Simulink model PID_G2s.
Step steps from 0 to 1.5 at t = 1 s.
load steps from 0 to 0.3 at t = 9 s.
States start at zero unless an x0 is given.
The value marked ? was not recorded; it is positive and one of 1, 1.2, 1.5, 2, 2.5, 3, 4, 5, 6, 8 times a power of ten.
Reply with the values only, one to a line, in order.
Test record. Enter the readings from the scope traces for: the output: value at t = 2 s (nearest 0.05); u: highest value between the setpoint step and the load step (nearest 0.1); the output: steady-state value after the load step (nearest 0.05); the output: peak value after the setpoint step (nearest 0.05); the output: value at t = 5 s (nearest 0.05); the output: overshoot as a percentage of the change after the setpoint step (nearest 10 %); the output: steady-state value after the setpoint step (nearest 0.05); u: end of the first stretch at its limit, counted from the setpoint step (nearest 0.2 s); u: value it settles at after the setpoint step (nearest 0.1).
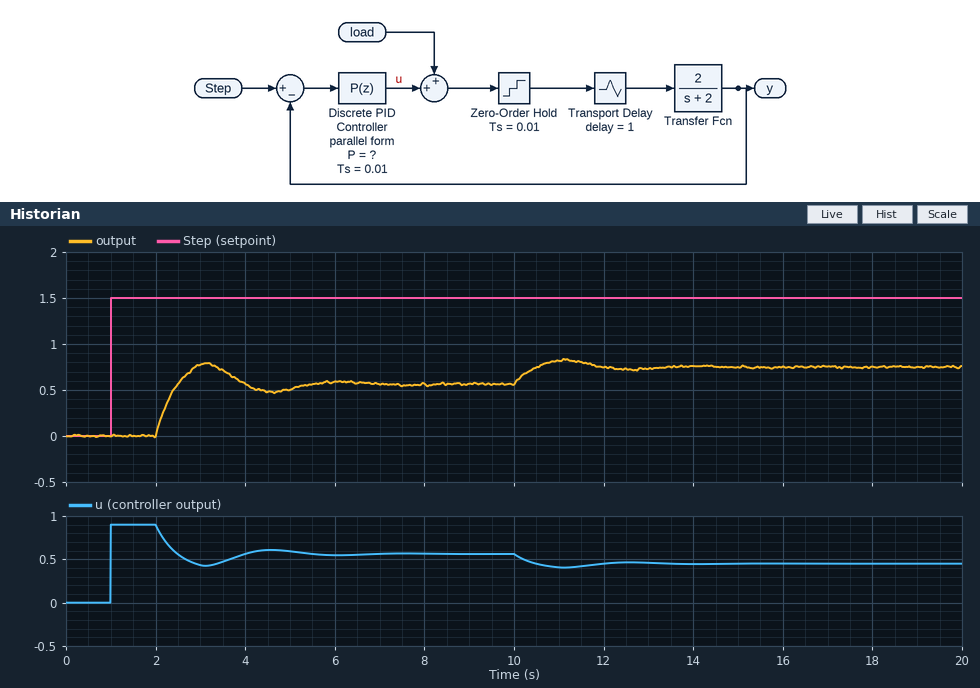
0.00
0.9
0.75
0.80
0.50
40 %
0.55
1.0 s
0.6
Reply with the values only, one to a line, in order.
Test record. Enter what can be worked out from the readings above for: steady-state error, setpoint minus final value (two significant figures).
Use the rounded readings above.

0.95
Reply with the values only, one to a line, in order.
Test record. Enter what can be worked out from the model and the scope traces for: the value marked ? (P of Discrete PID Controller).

0.6
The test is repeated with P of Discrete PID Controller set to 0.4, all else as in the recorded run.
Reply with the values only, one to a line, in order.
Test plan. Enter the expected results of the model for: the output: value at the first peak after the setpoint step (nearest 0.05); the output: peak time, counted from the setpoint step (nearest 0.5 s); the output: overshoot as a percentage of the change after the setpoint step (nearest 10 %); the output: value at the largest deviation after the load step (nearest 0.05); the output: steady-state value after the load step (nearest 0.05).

0.55
2.0 s
20 %
0.70
0.65
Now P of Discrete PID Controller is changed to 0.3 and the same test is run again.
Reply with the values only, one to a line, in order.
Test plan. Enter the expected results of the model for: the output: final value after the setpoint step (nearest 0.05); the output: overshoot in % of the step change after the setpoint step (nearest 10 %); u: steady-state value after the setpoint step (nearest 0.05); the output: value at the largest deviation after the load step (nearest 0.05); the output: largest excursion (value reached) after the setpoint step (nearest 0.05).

0.35
20 %
0.35
0.60
0.40
